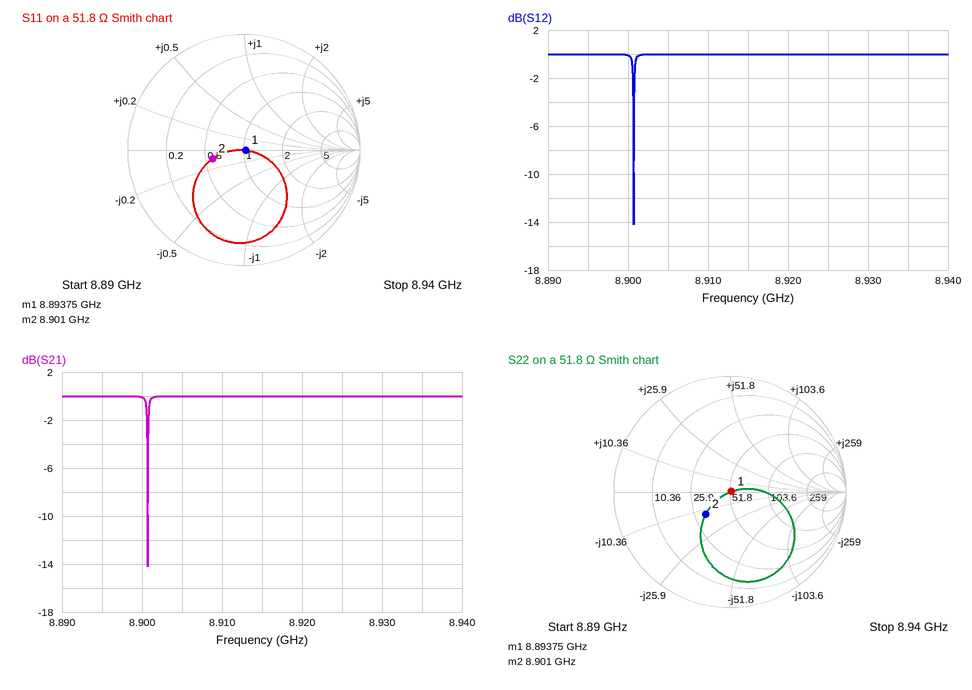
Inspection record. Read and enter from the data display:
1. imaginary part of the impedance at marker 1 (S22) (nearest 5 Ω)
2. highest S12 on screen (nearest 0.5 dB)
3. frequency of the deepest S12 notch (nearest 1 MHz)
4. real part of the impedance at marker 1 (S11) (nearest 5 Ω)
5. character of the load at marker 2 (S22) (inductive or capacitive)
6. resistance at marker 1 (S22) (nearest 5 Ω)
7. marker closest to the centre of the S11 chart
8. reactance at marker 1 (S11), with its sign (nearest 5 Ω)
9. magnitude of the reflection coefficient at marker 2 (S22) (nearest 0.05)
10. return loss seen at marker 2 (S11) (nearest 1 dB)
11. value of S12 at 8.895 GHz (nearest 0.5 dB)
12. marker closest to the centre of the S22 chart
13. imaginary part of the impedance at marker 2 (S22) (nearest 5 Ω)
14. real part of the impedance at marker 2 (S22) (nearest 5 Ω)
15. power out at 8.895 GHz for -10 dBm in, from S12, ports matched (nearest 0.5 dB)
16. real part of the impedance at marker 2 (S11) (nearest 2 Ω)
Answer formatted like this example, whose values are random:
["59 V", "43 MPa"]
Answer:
["0 Ω", "0.0 dB", "8.901 GHz", "55 Ω", "capacitive", "55 Ω", "marker 1", "0 Ω", "0.30", "11 dB", "0.0 dB", "marker 1", "-15 Ω", "30 Ω", "-10.0 dBm", "30 Ω"]
